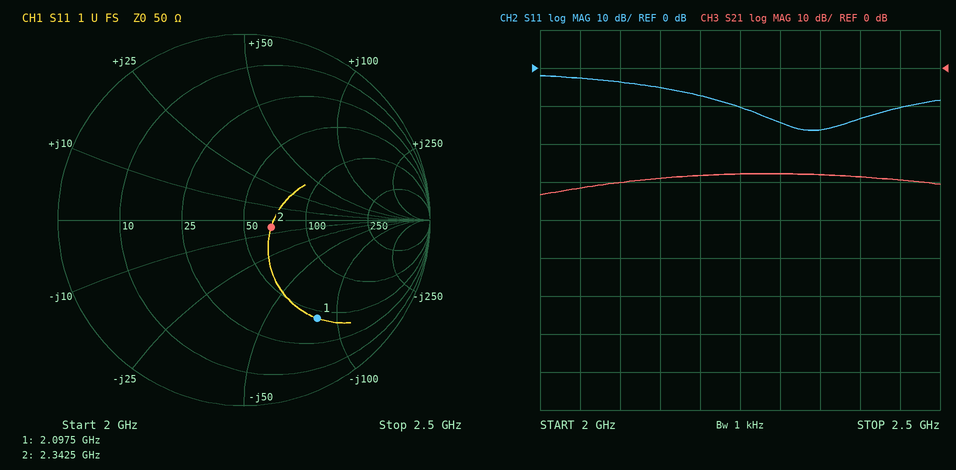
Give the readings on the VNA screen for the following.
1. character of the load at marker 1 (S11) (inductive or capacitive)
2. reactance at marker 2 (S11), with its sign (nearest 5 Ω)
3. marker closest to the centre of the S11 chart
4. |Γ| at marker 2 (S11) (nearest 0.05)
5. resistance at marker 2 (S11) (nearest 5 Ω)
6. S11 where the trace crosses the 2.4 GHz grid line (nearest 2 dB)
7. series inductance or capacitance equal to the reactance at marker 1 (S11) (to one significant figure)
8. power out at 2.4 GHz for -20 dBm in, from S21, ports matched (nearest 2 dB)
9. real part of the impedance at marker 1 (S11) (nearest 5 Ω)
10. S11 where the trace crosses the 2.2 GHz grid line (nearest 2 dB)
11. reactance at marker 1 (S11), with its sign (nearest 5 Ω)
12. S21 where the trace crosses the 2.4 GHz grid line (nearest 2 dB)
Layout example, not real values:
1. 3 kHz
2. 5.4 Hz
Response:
1. capacitive
2. -5 Ω
3. marker 2
4. 0.15
5. 65 Ω
6. -14 dB
7. 900 fF
8. -48 dBm
9. 45 Ω
10. -8 dB
11. -80 Ω
12. -28 dB
